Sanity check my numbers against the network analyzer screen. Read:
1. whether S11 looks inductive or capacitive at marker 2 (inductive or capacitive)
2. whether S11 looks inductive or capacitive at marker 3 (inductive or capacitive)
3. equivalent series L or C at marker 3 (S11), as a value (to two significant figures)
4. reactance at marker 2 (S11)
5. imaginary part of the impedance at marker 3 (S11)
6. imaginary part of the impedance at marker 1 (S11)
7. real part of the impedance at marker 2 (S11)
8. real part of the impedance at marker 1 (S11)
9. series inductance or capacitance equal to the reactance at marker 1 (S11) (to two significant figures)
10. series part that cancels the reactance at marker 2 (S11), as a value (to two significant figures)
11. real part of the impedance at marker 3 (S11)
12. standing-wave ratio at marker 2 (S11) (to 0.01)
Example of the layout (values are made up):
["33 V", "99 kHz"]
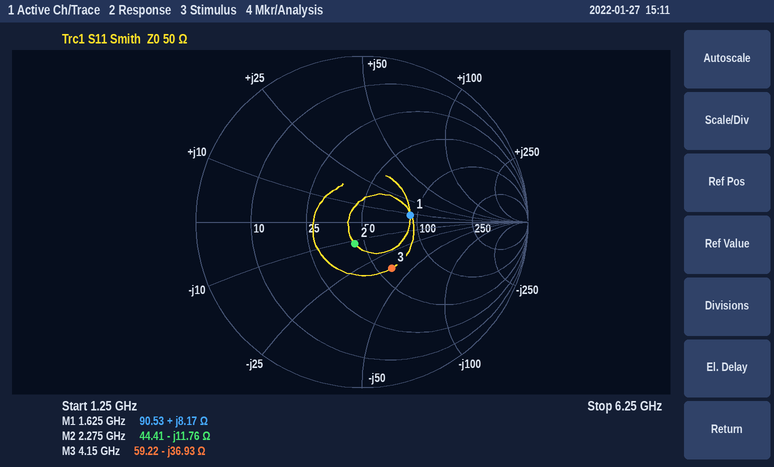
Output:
["capacitive", "capacitive", "1.0 pF", "-11.76 Ω", "-36.93 Ω", "+8.17 Ω", "44.41 Ω", "90.53 Ω", "800 pH", "820 pH", "59.22 Ω", "1.32"]
